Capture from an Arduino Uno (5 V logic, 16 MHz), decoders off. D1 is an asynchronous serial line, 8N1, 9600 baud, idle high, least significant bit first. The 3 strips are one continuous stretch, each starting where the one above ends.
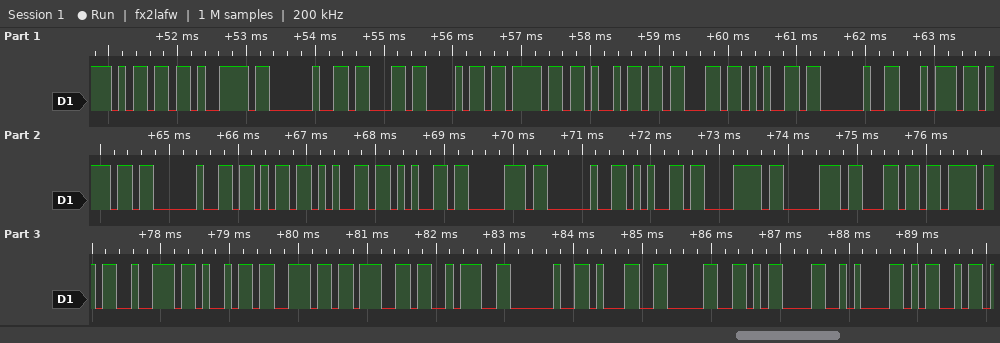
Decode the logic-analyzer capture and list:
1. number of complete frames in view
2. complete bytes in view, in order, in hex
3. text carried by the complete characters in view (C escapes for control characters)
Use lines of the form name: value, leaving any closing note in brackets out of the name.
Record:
number of complete frames in view: 34
complete bytes in view, in order, in hex: 6D 79 20 63 68 6F 69 63 65 20 74 6F 20 6B 65 65 70 20 65 78 70 6C 6F 72 69 6E 67 3A 20 31 30 0D 0A 4D
text carried by the complete characters in view: "my choice to keep exploring: 10\r\nM"
